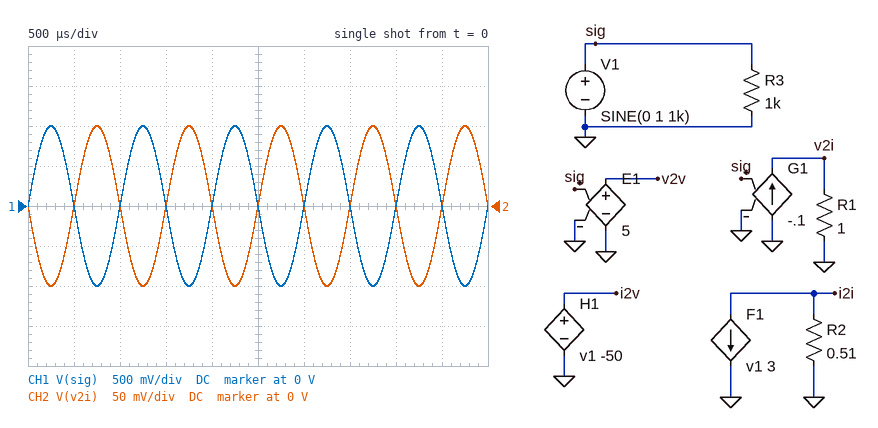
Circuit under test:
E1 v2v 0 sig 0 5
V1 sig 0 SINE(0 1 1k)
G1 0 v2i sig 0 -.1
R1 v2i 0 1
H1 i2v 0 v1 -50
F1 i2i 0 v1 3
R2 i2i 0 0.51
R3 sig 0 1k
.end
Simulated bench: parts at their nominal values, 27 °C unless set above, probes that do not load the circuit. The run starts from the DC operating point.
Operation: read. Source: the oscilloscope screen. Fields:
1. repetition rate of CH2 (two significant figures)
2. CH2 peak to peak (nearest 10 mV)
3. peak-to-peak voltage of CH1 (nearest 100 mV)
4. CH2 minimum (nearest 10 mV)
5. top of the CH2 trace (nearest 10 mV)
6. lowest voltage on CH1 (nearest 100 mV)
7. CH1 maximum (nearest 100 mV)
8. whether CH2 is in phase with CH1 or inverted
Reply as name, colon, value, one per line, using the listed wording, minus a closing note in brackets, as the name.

repetition rate of CH2: 1.0 kHz
CH2 peak to peak: 200 mV
peak-to-peak voltage of CH1: 2.0 V
CH2 minimum: -100 mV
top of the CH2 trace: 100 mV
lowest voltage on CH1: -1.0 V
CH1 maximum: 1.0 V
whether CH2 is in phase with CH1 or inverted: inverted
